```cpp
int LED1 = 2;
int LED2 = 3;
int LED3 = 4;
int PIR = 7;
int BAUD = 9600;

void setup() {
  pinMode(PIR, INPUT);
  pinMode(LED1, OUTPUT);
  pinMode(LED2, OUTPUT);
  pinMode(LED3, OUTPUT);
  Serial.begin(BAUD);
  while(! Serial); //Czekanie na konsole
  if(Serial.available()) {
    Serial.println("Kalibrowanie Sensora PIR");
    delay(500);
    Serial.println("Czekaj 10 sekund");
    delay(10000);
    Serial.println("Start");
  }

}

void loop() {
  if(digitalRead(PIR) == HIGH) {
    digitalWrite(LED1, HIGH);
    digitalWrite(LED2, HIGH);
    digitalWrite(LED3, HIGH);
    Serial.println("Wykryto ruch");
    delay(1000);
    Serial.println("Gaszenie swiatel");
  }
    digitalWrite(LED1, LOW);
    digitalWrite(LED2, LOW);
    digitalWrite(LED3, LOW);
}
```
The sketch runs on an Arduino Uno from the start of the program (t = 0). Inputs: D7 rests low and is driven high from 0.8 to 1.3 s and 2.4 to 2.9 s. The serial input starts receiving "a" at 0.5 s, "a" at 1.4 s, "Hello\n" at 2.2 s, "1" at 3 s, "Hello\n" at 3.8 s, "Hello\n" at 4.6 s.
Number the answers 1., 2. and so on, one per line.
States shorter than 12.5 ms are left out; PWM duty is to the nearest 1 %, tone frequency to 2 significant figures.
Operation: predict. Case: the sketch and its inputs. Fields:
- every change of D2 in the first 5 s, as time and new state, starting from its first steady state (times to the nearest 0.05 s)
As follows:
1. 0 s low; 0.8 s high; 1.8 s low; 2.4 s high; 3.4 s low
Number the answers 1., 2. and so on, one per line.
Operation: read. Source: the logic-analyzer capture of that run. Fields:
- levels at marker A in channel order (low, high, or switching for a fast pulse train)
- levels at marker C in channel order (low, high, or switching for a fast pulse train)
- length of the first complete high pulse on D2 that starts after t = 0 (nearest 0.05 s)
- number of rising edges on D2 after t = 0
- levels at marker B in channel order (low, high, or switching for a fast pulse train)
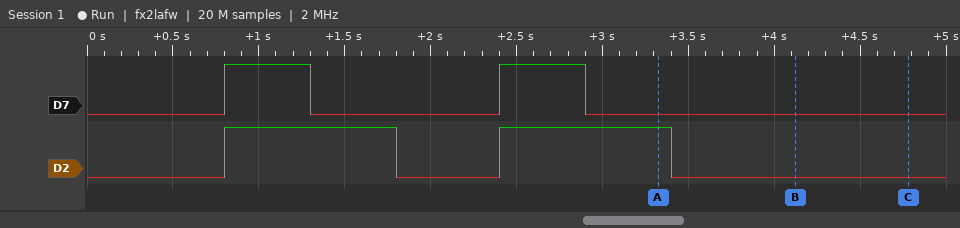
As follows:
1. D7 low, D2 high
2. D7 low, D2 low
3. 1.00 s
4. 2
5. D7 low, D2 low
